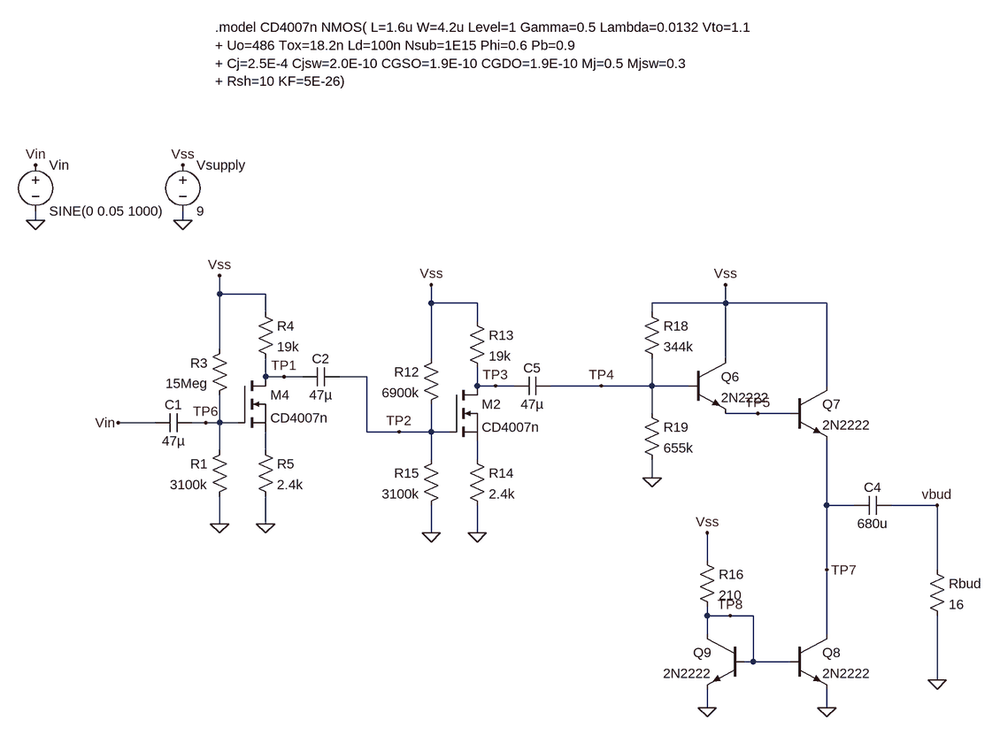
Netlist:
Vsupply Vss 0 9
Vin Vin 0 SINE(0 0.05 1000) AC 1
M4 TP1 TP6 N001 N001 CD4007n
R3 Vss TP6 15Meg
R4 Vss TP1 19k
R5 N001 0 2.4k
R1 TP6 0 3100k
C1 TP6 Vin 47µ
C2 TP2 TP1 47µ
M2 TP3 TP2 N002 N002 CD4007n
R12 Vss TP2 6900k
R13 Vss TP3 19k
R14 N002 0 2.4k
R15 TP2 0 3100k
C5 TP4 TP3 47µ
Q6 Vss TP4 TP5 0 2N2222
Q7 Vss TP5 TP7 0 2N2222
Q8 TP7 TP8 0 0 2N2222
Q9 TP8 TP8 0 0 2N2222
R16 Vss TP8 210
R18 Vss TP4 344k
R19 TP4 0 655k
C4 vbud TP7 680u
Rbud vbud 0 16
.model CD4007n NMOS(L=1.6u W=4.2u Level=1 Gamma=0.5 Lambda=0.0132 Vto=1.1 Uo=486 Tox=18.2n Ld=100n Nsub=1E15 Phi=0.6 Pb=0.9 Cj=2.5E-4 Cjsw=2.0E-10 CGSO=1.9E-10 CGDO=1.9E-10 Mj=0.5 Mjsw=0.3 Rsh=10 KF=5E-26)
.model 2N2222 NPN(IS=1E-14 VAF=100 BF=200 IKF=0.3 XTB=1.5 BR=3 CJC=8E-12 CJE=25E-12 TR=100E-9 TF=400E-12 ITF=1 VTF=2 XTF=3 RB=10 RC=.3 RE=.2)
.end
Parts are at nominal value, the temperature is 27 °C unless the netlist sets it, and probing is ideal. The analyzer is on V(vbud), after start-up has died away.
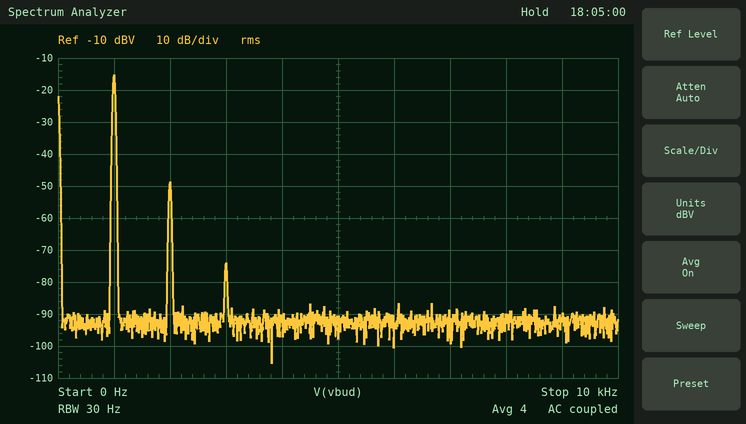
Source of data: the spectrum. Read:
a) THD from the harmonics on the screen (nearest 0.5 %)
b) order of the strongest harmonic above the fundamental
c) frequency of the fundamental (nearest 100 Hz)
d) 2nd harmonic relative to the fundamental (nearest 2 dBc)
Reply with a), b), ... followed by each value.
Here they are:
a) 2.0 %
b) 2
c) 1.0 kHz
d) -34 dBc
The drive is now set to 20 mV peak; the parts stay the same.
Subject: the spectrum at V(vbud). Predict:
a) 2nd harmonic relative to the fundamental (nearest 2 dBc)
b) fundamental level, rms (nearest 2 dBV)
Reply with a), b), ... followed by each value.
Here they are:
a) -42 dBc
b) -24 dBV
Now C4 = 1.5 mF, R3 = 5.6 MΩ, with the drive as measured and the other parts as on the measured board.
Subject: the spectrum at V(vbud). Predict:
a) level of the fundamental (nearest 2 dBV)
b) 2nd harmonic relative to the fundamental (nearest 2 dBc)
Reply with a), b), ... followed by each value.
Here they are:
a) -8 dBV
b) -38 dBc
